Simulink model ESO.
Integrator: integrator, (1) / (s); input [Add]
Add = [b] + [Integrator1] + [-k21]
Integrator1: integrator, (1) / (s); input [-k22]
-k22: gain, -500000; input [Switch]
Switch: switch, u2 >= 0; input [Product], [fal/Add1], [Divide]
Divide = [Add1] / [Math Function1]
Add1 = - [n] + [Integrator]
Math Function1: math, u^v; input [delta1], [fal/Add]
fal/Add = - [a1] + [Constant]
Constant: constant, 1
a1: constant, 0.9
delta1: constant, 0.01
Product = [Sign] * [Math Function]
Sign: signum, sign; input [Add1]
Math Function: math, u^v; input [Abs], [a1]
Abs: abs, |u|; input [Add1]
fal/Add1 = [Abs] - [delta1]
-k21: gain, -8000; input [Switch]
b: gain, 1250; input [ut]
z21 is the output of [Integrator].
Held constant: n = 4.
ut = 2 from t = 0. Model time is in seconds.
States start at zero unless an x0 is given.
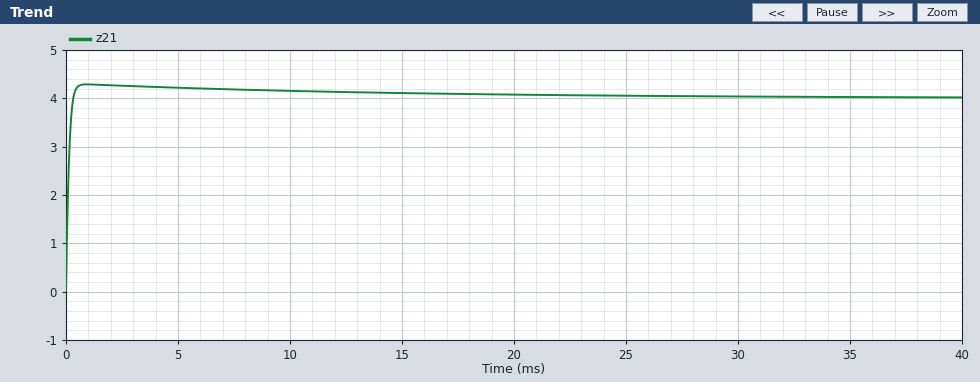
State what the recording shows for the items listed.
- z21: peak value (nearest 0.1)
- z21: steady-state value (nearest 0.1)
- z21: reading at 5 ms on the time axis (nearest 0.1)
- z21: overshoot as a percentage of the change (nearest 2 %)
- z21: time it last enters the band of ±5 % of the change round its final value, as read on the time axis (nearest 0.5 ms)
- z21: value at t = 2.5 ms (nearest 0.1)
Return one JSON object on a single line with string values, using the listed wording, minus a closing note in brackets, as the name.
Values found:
{"z21: peak value": "4.3", "z21: steady-state value": "4.0", "z21: reading at 5 ms on the time axis": "4.2", "z21: overshoot as a percentage of the change": "8 %", "z21: time it last enters the band of ±5 % of the change round its final value, as read on the time axis": "6.5 ms", "z21: value at t = 2.5 ms": "4.3"}
